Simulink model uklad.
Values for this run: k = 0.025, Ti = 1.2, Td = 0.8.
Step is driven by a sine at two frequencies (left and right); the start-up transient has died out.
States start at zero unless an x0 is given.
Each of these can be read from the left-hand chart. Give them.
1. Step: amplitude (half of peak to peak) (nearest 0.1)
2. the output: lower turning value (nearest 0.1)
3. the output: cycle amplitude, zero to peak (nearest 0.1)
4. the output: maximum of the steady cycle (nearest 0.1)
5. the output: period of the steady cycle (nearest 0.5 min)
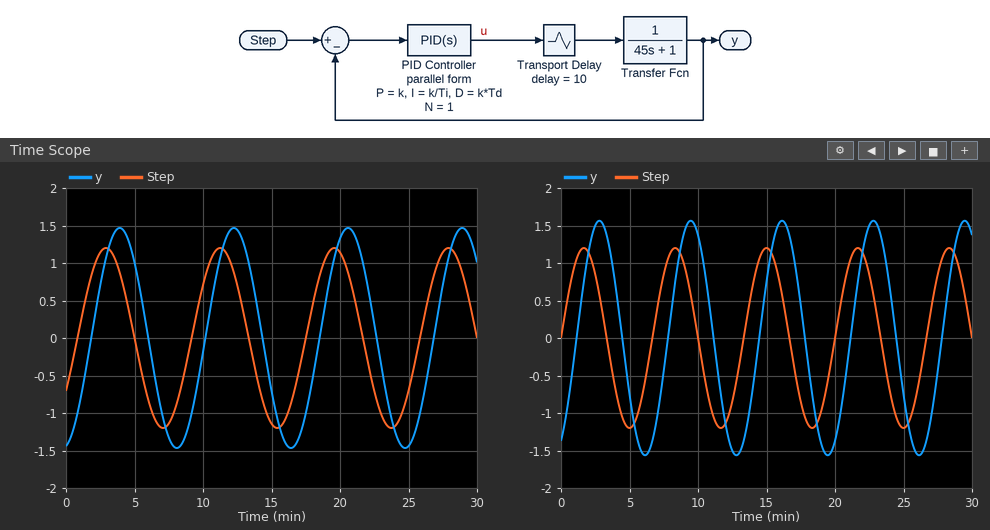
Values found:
1.2
-1.5
1.5
1.5
8.5 min
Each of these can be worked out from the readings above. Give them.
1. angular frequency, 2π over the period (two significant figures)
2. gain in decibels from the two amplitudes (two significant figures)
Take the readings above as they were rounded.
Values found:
0.74 rad/min
1.9 dB
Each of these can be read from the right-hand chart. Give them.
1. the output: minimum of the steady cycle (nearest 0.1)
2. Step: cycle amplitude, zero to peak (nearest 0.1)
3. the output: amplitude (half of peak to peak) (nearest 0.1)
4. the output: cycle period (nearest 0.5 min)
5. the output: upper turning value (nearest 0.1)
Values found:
-1.6
1.2
1.6
6.5 min
1.6
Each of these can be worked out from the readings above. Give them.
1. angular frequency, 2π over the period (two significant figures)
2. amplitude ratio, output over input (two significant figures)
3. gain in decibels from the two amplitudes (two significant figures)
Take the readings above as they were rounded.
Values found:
0.97 rad/min
1.3
2.5 dB
